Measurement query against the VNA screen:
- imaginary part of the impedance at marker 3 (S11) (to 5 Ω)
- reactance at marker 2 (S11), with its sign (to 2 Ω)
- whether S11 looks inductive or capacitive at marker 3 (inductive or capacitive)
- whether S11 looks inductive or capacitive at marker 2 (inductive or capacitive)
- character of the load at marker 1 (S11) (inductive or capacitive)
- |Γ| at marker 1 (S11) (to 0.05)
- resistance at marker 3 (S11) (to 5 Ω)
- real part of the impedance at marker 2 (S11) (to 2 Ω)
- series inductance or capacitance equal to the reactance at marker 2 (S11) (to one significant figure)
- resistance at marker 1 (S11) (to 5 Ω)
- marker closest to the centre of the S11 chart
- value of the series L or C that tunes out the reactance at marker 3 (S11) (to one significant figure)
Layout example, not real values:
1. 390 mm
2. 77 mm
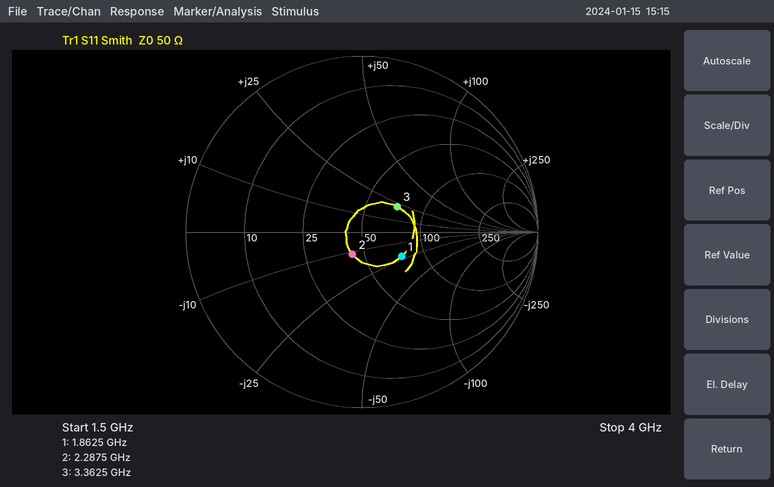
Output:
1. +20 Ω
2. -12 Ω
3. inductive
4. capacitive
5. capacitive
6. 0.25
7. 70 Ω
8. 44 Ω
9. 6 pF
10. 75 Ω
11. marker 2
12. 2 pF
